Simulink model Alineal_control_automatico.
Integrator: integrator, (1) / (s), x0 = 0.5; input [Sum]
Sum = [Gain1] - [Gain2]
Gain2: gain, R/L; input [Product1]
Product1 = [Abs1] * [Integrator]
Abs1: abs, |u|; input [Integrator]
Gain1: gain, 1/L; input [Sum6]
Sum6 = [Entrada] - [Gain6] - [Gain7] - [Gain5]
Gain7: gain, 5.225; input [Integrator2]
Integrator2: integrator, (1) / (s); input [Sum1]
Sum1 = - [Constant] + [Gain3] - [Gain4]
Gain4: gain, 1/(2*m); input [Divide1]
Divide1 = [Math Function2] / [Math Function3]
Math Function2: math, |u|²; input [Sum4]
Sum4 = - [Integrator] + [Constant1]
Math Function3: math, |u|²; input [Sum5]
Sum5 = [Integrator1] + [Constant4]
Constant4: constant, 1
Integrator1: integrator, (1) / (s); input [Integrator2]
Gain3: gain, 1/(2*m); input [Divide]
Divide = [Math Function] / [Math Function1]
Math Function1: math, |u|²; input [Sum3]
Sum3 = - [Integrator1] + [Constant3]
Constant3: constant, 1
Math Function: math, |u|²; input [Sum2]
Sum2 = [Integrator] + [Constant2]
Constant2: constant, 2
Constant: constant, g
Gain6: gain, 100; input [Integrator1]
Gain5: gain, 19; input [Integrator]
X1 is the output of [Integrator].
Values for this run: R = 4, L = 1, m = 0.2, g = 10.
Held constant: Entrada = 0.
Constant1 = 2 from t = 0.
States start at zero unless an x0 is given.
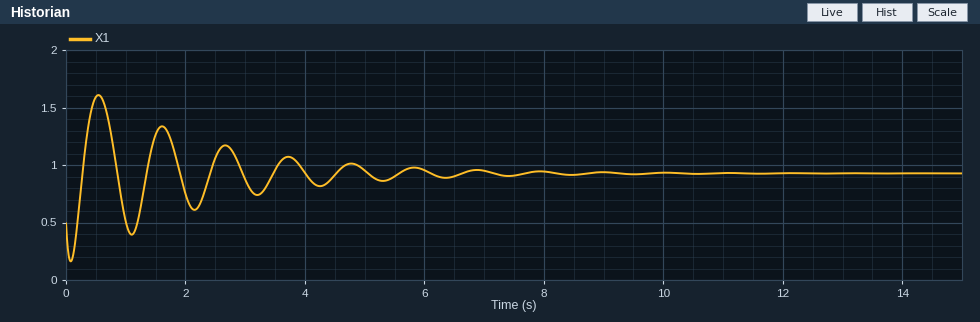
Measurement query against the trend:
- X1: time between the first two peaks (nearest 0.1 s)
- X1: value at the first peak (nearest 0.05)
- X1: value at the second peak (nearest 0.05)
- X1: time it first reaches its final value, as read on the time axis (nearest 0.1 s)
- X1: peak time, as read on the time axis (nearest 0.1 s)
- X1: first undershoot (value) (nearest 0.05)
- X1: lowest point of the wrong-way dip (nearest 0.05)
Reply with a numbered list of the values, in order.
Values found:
1. 1.1 s
2. 1.60
3. 1.35
4. 0.3 s
5. 0.5 s
6. 0.40
7. 0.15
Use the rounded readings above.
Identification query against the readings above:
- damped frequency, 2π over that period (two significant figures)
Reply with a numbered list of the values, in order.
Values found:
1. 5.7 rad/s
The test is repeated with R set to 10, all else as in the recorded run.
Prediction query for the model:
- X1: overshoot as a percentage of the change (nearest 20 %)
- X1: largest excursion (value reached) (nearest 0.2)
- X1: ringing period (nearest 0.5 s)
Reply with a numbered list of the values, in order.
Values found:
1. 80 %
2. 2.0
3. 2.0 s
